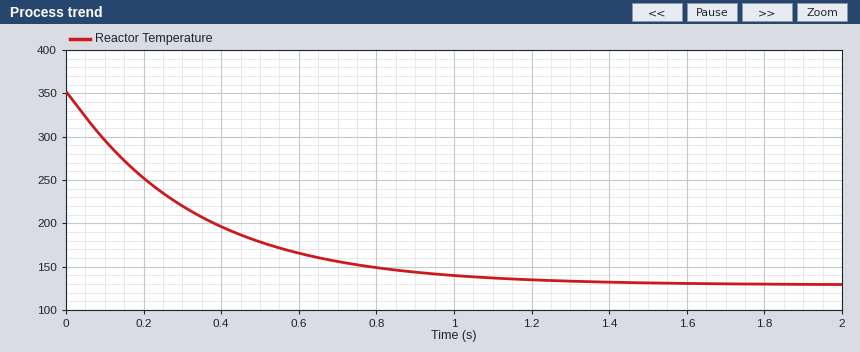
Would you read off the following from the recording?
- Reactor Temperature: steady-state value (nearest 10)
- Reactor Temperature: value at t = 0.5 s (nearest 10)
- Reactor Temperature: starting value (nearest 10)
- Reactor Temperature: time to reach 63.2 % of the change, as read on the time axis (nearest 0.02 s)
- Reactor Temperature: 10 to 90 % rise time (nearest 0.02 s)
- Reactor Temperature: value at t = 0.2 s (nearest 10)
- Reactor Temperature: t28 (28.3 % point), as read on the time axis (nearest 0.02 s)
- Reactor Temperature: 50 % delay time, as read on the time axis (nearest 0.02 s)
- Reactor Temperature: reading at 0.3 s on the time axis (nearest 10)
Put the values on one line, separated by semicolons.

130; 180; 350; 0.34 s; 0.72 s; 250; 0.12 s; 0.24 s; 220
